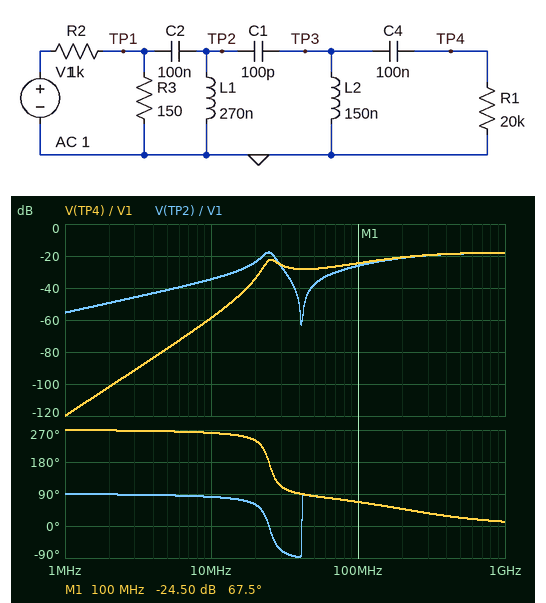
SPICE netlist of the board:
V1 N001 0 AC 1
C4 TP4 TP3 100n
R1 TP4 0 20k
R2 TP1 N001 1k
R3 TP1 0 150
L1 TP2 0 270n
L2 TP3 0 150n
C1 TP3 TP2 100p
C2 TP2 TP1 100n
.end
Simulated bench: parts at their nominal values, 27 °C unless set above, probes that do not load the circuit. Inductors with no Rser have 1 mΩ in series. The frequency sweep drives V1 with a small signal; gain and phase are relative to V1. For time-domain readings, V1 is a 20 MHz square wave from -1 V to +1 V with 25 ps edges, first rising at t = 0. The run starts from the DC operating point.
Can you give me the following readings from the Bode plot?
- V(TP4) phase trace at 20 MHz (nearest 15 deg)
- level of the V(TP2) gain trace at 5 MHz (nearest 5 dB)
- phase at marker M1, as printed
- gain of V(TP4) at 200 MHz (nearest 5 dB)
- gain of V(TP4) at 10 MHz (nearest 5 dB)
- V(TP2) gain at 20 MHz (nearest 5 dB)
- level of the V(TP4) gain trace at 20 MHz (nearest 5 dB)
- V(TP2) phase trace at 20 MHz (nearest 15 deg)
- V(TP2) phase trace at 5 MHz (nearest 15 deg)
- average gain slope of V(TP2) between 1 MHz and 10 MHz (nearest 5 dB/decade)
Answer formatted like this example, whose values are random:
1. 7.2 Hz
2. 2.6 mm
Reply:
1. 240 deg
2. -40 dB
3. 67.5 deg
4. -20 dB
5. -60 dB
6. -25 dB
7. -35 dB
8. 60 deg
9. 90 deg
10. 20 dB/decade
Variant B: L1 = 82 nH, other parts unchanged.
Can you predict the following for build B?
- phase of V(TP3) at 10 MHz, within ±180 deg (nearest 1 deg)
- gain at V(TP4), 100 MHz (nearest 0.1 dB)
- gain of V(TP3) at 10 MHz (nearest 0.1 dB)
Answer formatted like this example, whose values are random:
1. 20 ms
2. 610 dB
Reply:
1. -92 deg
2. -28.8 dB
3. -69.5 dB
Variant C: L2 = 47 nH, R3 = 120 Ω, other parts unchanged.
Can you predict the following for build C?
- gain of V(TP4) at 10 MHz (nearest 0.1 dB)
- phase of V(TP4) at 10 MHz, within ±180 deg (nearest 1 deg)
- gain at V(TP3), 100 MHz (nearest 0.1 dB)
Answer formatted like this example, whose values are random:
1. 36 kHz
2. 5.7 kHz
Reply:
1. -69.0 dB
2. -100 deg
3. -31.3 dB
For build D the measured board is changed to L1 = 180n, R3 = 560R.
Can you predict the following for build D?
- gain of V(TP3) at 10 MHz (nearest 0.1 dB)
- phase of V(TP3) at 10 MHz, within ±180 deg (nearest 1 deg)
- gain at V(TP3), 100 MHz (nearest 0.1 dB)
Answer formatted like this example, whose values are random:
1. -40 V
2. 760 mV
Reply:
1. -62.3 dB
2. -92 deg
3. -25.2 dB
